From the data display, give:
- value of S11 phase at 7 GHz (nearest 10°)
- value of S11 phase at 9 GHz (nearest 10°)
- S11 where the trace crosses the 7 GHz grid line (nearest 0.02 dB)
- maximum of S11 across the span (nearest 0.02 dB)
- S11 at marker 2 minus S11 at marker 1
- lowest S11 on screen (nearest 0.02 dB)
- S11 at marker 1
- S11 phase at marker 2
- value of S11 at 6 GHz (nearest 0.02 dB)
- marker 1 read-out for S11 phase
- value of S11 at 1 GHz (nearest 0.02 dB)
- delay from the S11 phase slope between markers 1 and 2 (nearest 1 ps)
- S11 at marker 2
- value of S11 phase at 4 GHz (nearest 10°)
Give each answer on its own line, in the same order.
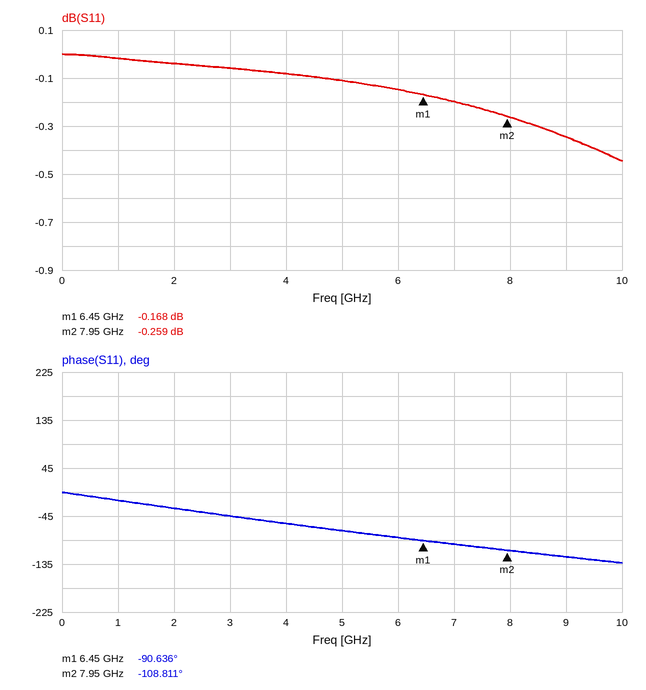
-100°
-120°
-0.20 dB
0.00 dB
-0.091 dB
-0.44 dB
-0.168 dB
-108.811°
-0.14 dB
-90.636°
-0.02 dB
34 ps
-0.259 dB
-60°
